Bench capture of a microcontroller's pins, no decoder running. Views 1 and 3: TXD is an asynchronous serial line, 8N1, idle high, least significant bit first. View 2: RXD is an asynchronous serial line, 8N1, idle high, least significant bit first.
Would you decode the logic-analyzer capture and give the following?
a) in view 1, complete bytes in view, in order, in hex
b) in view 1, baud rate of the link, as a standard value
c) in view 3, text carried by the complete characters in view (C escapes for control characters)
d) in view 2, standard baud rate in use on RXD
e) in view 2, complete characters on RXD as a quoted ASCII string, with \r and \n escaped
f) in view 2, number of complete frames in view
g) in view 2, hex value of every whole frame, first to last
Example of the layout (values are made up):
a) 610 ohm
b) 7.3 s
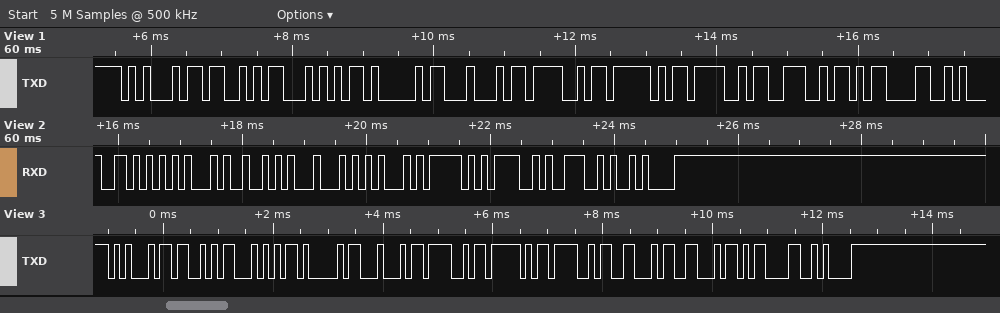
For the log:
a) 45 53 54 41 44 4F 5F 4F 4E 0D
b) 9600 baud
c) "ESTADO_OFF\r\n"
d) 9600 baud
e) "VERDE_ON\n"
f) 9
g) 56 45 52 44 45 5F 4F 4E 0A
